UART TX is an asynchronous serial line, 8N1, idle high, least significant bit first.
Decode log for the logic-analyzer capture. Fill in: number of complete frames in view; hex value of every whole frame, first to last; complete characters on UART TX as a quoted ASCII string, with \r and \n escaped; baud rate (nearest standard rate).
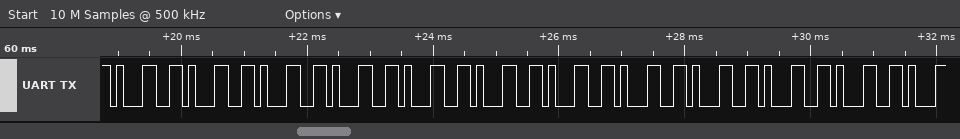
11
0x31 0x31 0x31 0x31 0x31 0x31 0x31 0x31 0x31 0x31 0x31
"11111111111"
9600 baud
